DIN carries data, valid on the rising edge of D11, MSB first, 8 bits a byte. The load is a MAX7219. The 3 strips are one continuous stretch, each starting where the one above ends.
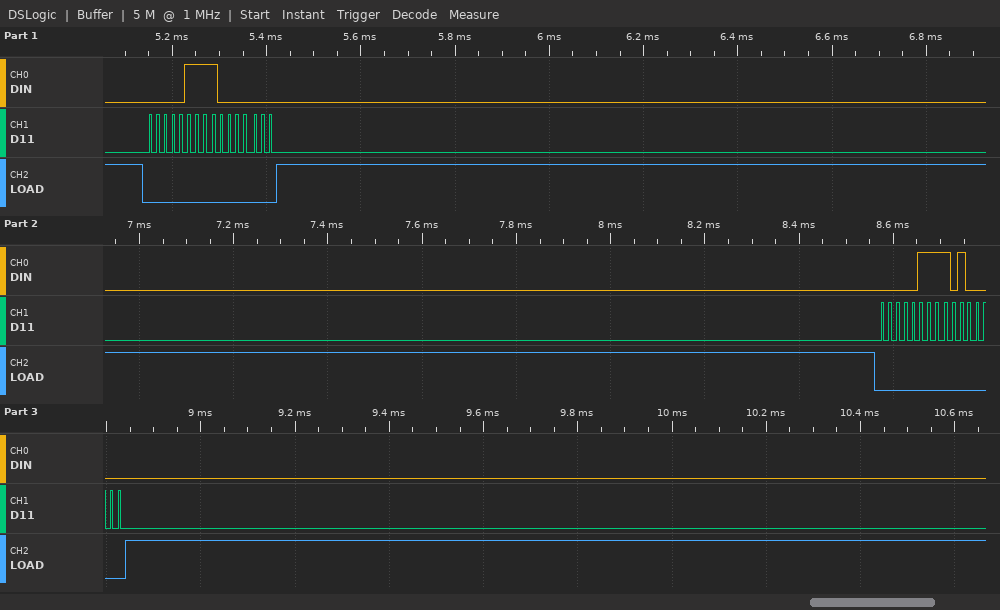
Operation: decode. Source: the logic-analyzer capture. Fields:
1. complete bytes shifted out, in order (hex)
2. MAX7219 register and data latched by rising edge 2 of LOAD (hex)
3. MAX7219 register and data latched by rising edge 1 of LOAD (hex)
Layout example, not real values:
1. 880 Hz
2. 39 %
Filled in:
1. 07 80 07 A0
2. register 0x7, data 0xA0
3. register 0x7, data 0x80
